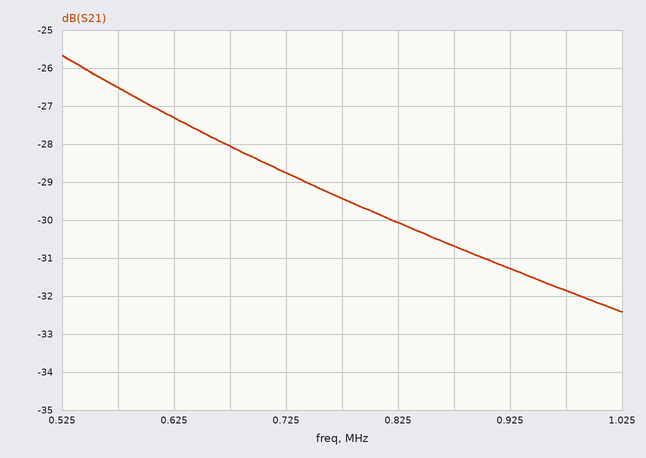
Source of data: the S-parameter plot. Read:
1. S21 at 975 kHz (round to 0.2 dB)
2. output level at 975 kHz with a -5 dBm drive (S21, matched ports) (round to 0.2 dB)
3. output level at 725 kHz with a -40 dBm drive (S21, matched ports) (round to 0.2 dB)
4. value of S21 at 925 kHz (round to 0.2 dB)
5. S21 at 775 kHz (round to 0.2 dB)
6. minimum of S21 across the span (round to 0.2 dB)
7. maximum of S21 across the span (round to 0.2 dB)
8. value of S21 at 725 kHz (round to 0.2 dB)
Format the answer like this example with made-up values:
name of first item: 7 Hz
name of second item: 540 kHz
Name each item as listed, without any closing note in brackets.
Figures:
S21 at 975 kHz: -31.8 dB
output level at 975 kHz with a -5 dBm drive (S21, matched ports): -36.8 dBm
output level at 725 kHz with a -40 dBm drive (S21, matched ports): -68.8 dBm
value of S21 at 925 kHz: -31.2 dB
S21 at 775 kHz: -29.4 dB
minimum of S21 across the span: -32.4 dB
maximum of S21 across the span: -25.6 dB
value of S21 at 725 kHz: -28.8 dB
